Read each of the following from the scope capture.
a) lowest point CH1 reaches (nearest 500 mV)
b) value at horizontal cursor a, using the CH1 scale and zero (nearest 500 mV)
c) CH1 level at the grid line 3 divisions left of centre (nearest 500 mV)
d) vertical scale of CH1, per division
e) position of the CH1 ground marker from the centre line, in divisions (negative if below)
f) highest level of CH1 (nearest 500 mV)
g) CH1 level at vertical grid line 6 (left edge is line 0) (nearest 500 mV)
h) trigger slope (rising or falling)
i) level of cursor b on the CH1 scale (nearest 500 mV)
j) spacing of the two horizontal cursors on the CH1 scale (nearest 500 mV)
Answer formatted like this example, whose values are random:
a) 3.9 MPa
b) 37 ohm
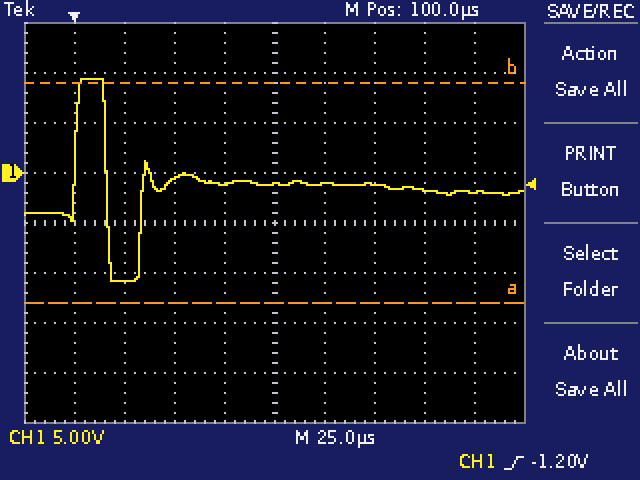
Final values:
a) -11.0 V
b) -13.0 V
c) -11.0 V
d) 5 V
e) +1.0 div
f) 9.5 V
g) -1.0 V
h) rising
i) 9.0 V
j) 22.0 V
